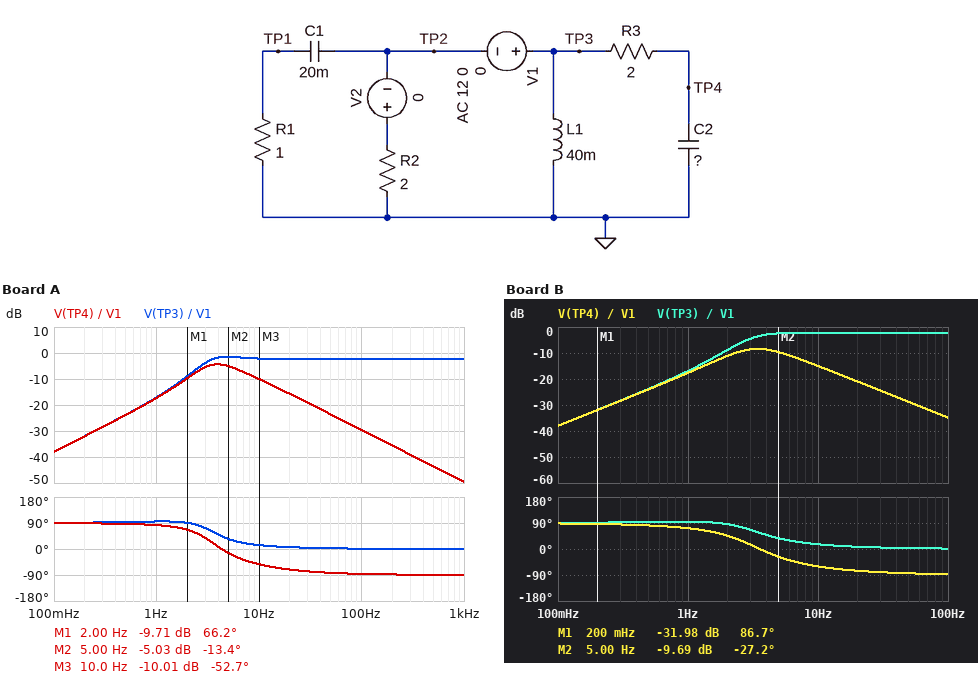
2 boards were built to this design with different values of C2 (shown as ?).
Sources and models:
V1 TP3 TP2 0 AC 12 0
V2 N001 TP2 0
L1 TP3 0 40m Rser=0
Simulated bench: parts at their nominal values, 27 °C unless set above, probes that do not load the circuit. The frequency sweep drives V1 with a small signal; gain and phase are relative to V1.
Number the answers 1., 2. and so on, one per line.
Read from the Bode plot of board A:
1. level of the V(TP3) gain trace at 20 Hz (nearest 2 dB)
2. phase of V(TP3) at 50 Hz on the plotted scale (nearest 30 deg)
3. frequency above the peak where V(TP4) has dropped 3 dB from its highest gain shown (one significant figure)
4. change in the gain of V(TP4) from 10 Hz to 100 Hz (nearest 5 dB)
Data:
1. -2 dB
2. 0 deg
3. 7 Hz
4. -20 dB
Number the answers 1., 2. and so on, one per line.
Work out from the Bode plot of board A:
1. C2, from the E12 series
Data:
1. 18 mF
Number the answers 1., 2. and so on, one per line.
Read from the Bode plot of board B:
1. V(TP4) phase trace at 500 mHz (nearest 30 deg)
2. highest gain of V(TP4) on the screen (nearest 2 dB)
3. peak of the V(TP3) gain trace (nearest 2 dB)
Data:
1. 90 deg
2. -8 dB
3. -2 dB
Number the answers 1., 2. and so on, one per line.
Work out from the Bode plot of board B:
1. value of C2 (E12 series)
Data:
1. 33 mF
